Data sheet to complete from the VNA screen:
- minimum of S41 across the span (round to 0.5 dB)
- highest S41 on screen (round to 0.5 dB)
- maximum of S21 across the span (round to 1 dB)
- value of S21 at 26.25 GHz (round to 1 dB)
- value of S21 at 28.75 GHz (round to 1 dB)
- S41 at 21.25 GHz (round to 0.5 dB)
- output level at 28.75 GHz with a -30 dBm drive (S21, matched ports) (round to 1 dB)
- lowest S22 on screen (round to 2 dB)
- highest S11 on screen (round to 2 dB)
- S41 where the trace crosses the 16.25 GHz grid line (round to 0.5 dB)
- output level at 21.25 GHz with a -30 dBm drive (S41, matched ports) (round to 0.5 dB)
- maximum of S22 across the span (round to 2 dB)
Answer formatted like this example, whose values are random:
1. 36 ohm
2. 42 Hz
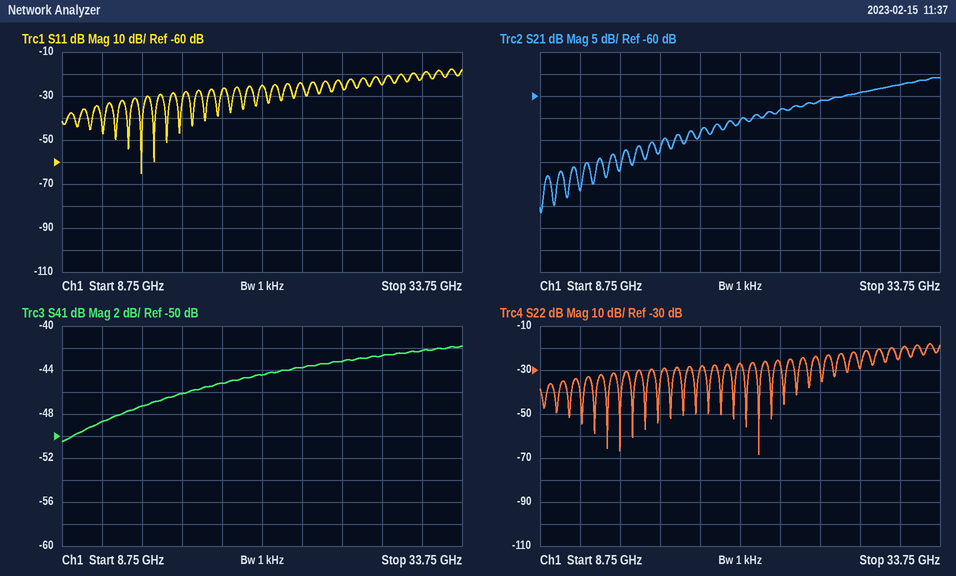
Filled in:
1. -50.5 dB
2. -42.0 dB
3. -56 dB
4. -61 dB
5. -59 dB
6. -44.5 dB
7. -89 dBm
8. -68 dB
9. -18 dB
10. -46.0 dB
11. -74.5 dBm
12. -18 dB
